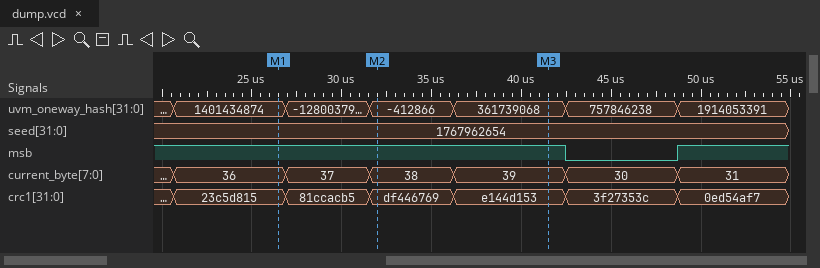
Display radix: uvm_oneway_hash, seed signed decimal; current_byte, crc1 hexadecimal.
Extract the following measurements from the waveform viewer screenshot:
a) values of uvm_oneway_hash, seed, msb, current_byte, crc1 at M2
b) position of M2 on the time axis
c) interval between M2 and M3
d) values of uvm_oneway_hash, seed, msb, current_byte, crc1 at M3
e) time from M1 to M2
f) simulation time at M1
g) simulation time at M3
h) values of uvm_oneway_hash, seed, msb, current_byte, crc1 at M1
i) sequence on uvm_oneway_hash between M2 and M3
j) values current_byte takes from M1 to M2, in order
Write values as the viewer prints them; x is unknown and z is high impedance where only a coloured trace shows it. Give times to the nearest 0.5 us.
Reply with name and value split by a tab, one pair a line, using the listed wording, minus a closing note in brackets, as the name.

values of uvm_oneway_hash, seed, msb, current_byte, crc1 at M2	uvm_oneway_hash=-412866, seed=1767962654, msb=1, current_byte=38, crc1=df446769
position of M2 on the time axis	32 us
interval between M2 and M3	9.5 us
values of uvm_oneway_hash, seed, msb, current_byte, crc1 at M3	uvm_oneway_hash=361739068, seed=1767962654, msb=1, current_byte=39, crc1=e144d153
time from M1 to M2	5.5 us
simulation time at M1	26.5 us
simulation time at M3	41.5 us
values of uvm_oneway_hash, seed, msb, current_byte, crc1 at M1	uvm_oneway_hash=1401434874, seed=1767962654, msb=1, current_byte=36, crc1=23c5d815
sequence on uvm_oneway_hash between M2 and M3	-412866, 361739068
values current_byte takes from M1 to M2, in order	36, 37, 38
